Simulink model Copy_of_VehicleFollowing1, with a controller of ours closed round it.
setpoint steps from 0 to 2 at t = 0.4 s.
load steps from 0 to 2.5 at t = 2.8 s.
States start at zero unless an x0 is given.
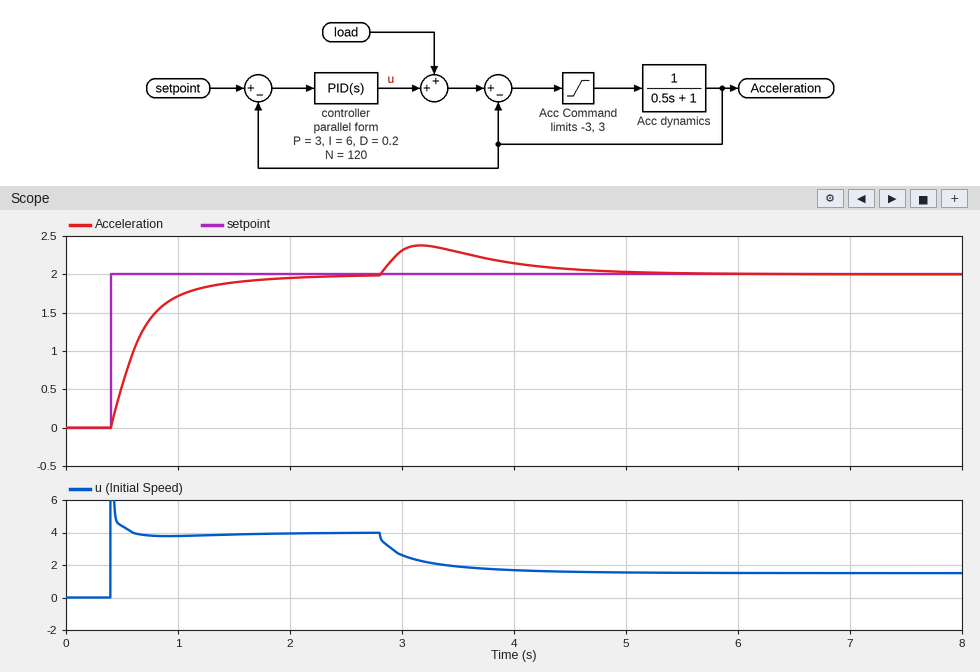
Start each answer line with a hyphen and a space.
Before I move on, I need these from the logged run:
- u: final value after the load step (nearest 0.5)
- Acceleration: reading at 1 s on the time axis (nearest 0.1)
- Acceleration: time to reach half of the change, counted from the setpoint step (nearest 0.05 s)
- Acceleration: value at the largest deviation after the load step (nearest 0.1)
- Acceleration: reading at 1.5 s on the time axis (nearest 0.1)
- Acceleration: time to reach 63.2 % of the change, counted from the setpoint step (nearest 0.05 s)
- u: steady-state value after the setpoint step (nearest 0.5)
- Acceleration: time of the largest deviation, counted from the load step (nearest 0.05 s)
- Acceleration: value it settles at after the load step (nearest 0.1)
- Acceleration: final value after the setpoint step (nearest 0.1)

- 1.5
- 1.7
- 0.20 s
- 2.4
- 1.9
- 0.30 s
- 4.0
- 0.35 s
- 2.0
- 2.0
